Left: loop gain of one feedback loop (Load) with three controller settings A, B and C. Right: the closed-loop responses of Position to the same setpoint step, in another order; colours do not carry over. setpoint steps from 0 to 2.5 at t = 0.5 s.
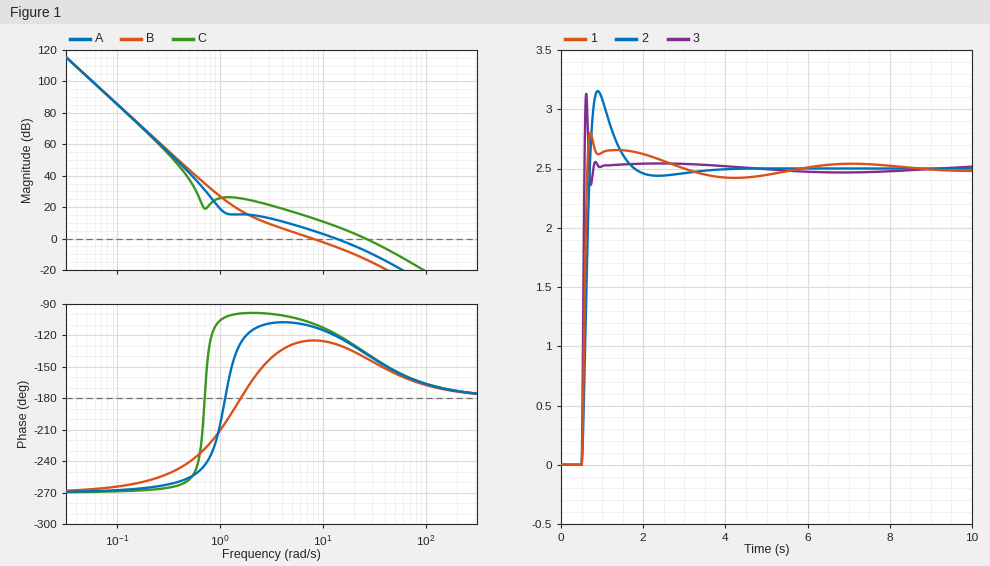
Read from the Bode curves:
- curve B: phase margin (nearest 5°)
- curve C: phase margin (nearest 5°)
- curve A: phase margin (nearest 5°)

55°
45°
60°
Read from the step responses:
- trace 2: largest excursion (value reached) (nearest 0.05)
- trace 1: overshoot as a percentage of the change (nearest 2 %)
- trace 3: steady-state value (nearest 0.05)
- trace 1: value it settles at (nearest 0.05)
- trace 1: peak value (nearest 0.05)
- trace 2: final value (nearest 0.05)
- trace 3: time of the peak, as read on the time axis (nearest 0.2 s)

3.15
12 %
2.50
2.50
2.80
2.50
0.6 s
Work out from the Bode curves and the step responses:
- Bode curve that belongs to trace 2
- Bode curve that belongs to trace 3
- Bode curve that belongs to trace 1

B
C
A
